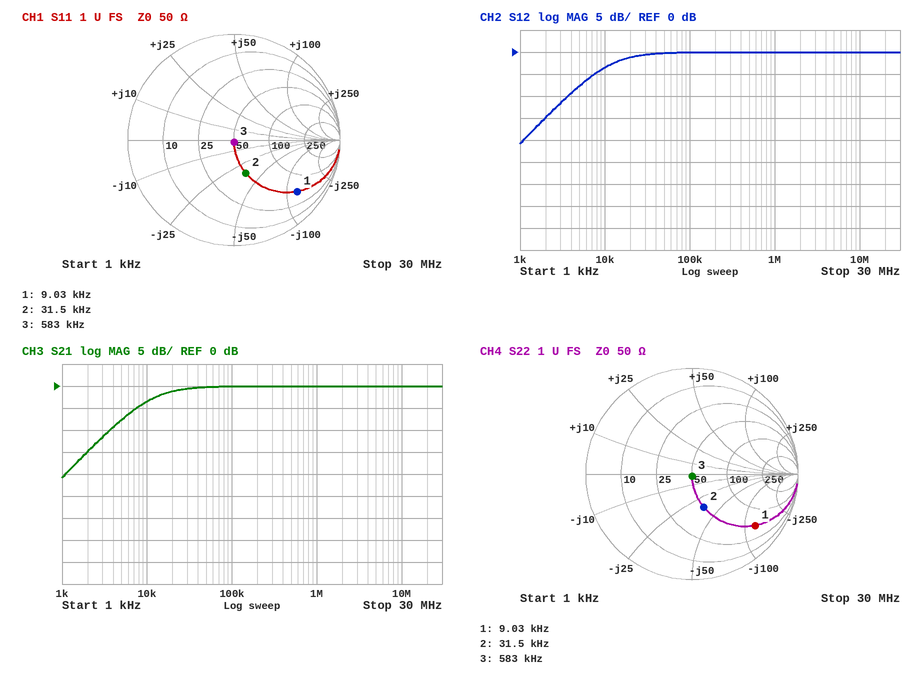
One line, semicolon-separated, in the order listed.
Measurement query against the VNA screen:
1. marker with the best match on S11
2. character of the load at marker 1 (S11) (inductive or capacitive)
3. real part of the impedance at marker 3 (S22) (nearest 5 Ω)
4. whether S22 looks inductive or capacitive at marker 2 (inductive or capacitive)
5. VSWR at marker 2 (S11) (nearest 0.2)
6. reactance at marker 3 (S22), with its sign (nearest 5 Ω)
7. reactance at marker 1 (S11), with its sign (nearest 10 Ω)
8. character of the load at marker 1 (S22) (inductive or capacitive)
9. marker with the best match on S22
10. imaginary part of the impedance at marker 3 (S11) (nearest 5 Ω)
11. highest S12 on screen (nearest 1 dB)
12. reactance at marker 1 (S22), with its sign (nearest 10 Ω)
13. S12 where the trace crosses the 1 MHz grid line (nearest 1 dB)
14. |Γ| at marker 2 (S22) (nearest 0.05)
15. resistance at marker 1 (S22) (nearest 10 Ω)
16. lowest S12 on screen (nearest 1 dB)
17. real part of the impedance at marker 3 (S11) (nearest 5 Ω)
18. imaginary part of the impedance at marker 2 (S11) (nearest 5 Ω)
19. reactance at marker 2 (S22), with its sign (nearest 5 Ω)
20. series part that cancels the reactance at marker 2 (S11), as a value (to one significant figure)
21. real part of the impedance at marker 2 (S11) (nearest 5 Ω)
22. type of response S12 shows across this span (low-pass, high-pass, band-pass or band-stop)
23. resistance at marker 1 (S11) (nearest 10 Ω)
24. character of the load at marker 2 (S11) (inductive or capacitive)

marker 3; capacitive; 50 Ω; capacitive; 2.0; 0 Ω; -120 Ω; capacitive; marker 3; 0 Ω; 0 dB; -120 Ω; 0 dB; 0.35; 50 Ω; -21 dB; 50 Ω; -35 Ω; -35 Ω; 200 µH; 50 Ω; high-pass; 50 Ω; capacitive
